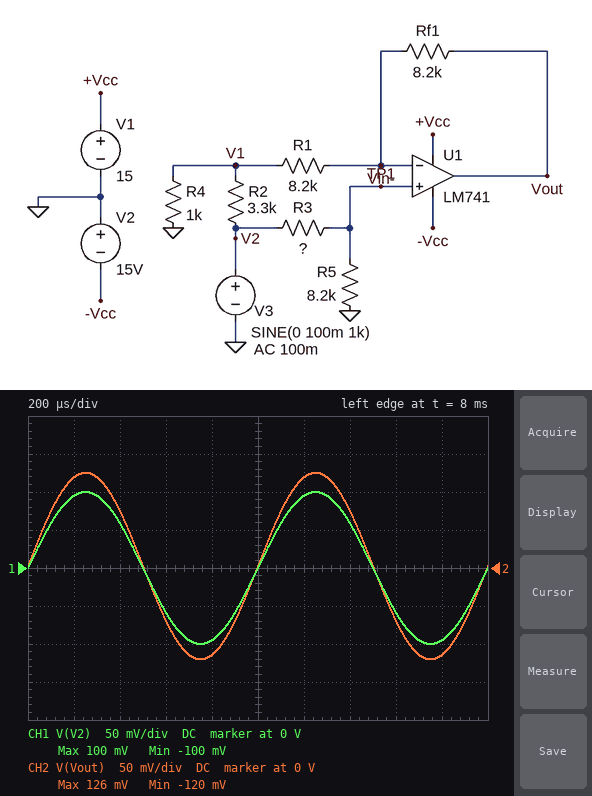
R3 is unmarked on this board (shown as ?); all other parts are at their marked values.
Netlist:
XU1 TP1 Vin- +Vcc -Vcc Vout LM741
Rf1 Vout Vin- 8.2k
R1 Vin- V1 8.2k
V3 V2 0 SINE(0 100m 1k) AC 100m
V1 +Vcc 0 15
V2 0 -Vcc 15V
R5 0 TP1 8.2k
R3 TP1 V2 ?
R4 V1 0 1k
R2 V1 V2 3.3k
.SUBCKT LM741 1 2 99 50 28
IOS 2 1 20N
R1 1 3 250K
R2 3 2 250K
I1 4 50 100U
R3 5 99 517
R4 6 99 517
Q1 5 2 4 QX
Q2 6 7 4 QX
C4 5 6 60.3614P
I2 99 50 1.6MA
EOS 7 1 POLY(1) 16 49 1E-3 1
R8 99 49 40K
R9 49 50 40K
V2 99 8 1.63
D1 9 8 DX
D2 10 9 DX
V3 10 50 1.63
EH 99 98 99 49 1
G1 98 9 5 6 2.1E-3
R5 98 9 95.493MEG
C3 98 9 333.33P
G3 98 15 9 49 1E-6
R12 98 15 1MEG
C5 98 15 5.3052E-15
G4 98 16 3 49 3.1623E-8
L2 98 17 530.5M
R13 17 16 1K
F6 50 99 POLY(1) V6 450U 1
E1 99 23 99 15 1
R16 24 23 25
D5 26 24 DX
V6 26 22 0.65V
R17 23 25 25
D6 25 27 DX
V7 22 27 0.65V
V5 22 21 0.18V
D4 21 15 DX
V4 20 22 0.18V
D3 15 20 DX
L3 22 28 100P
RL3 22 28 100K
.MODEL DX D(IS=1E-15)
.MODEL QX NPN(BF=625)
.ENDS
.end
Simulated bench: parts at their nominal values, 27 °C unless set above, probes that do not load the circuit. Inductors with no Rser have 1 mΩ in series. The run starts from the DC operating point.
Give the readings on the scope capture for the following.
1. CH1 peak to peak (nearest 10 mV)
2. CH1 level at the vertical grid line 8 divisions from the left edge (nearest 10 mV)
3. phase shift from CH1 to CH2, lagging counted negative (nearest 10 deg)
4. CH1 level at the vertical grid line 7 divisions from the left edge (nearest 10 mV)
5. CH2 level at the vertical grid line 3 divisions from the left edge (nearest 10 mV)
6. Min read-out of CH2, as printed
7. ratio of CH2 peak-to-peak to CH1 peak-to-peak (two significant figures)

200 mV
-60 mV
0 deg
60 mV
-70 mV
-120 mV
1.2
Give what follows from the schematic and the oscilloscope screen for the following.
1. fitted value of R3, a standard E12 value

2.7 kΩ
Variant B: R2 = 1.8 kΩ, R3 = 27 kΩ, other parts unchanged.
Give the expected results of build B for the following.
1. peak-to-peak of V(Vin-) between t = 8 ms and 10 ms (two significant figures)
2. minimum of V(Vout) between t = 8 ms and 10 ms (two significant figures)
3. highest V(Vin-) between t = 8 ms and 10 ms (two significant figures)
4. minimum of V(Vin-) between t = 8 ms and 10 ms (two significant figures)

47 mV
-9.7 mV
24 mV
-23 mV
